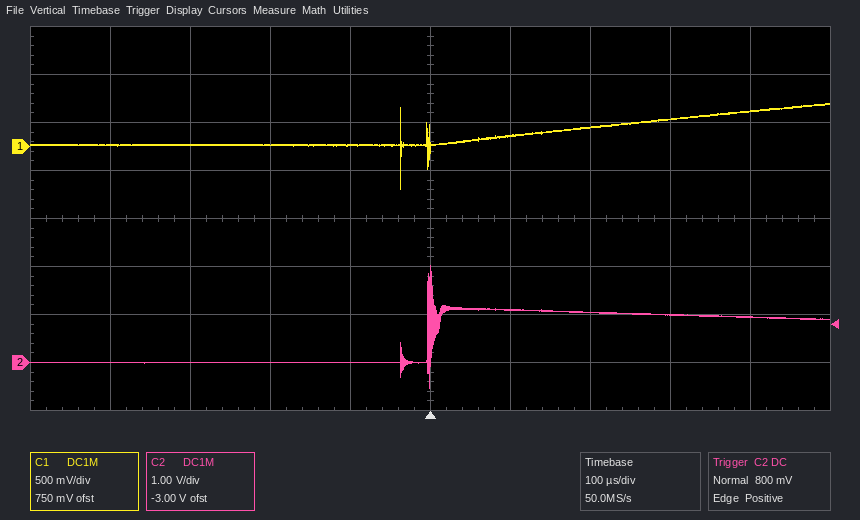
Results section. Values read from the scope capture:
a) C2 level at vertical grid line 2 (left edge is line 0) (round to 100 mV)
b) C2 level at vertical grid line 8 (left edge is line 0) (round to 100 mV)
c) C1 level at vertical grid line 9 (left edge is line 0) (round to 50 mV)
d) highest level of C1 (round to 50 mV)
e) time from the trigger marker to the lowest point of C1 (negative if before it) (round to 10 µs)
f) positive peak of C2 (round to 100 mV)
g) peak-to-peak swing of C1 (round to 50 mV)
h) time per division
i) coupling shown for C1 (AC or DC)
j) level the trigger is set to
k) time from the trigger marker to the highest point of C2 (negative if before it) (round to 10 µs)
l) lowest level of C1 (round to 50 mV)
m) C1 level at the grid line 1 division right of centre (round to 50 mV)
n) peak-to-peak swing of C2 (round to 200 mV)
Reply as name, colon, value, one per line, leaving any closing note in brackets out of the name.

C2 level at vertical grid line 2 (left edge is line 0): 0.0 V
C2 level at vertical grid line 8 (left edge is line 0): 1.0 V
C1 level at vertical grid line 9 (left edge is line 0): 350 mV
highest level of C1: 450 mV
time from the trigger marker to the lowest point of C1 (negative if before it): -40 µs
positive peak of C2: 2.0 V
peak-to-peak swing of C1: 900 mV
time per division: 100 µs
coupling shown for C1: DC
level the trigger is set to: 800 mV
time from the trigger marker to the highest point of C2 (negative if before it): 0 µs
lowest level of C1: -450 mV
C1 level at the grid line 1 division right of centre: 100 mV
peak-to-peak swing of C2: 2.6 V
